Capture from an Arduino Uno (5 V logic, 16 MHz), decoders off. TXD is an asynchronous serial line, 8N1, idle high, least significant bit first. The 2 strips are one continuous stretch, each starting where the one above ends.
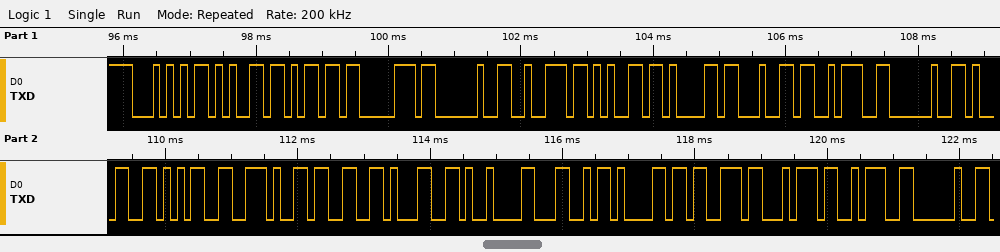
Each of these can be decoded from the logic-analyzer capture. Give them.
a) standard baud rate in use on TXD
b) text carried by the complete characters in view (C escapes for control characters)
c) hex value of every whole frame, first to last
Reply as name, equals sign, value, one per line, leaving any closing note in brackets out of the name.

standard baud rate in use on TXD = 9600 baud
text carried by the complete characters in view = "Temp read: 15.31\tLast: "
hex value of every whole frame, first to last = 54 65 6D 70 20 72 65 61 64 3A 20 31 35 2E 33 31 09 4C 61 73 74 3A 20
